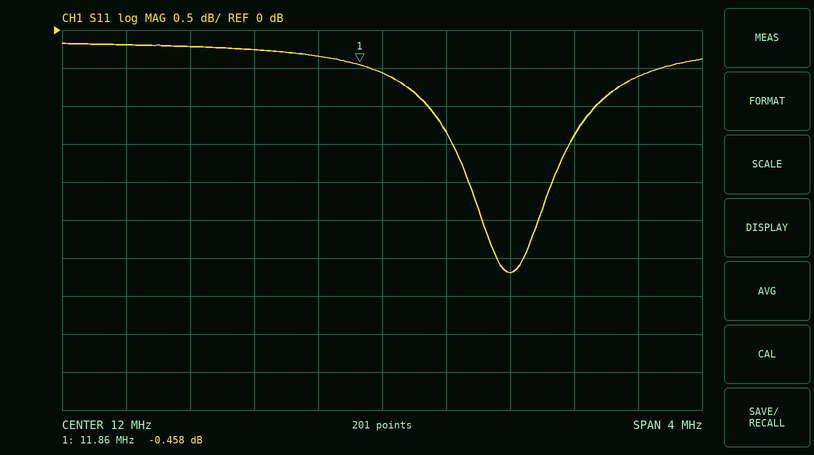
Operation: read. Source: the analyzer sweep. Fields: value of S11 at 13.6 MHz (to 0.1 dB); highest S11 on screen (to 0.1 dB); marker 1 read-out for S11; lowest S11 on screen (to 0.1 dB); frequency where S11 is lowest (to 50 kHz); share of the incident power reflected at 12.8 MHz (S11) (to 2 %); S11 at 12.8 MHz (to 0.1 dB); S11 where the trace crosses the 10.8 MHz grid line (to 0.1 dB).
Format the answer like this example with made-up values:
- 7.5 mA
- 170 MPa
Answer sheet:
- -0.6 dB
- -0.2 dB
- -0.458 dB
- -3.2 dB
- 12.80 MHz
- 48 %
- -3.2 dB
- -0.2 dB
